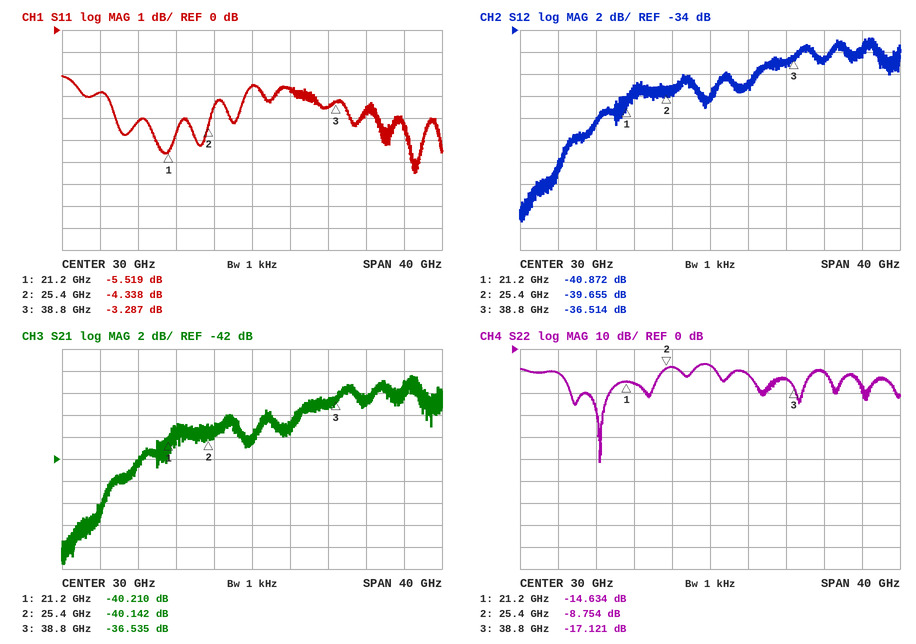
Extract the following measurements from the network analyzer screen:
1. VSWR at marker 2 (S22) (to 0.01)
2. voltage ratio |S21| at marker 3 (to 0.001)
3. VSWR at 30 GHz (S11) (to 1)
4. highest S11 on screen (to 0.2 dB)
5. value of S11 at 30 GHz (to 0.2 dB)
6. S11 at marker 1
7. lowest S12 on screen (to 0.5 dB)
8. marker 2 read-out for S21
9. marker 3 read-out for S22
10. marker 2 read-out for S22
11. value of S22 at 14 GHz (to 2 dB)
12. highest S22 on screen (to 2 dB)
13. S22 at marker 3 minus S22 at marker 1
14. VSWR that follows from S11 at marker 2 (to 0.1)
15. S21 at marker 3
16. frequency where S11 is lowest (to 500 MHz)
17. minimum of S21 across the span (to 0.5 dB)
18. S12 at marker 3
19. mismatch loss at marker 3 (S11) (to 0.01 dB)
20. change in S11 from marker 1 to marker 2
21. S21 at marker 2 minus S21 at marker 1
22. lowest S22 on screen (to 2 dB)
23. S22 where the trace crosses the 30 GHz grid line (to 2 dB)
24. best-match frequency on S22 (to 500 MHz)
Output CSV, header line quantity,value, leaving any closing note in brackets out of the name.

quantity,value
VSWR at marker 2 (S22),2.15
voltage ratio |S21| at marker 3,0.015
VSWR at 30 GHz (S11),7
highest S11 on screen,-2.0 dB
value of S11 at 30 GHz,-2.6 dB
S11 at marker 1,-5.519 dB
lowest S12 on screen,-51.5 dB
marker 2 read-out for S21,-40.142 dB
marker 3 read-out for S22,-17.121 dB
marker 2 read-out for S22,-8.754 dB
value of S22 at 14 GHz,-10 dB
highest S22 on screen,-6 dB
S22 at marker 3 minus S22 at marker 1,-2.487 dB
VSWR that follows from S11 at marker 2,4.1
S21 at marker 3,-36.535 dB
frequency where S11 is lowest,47.0 GHz
minimum of S21 across the span,-51.5 dB
S12 at marker 3,-36.514 dB
mismatch loss at marker 3 (S11),2.75 dB
change in S11 from marker 1 to marker 2,1.181 dB
S21 at marker 2 minus S21 at marker 1,0.068 dB
lowest S22 on screen,-52 dB
S22 where the trace crosses the 30 GHz grid line,-8 dB
best-match frequency on S22,18.5 GHz
